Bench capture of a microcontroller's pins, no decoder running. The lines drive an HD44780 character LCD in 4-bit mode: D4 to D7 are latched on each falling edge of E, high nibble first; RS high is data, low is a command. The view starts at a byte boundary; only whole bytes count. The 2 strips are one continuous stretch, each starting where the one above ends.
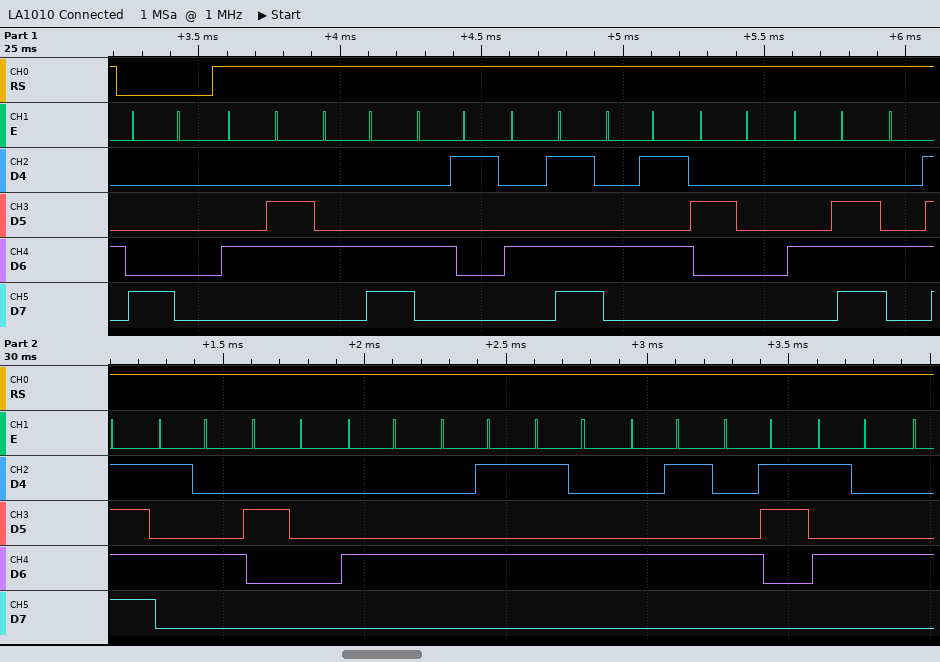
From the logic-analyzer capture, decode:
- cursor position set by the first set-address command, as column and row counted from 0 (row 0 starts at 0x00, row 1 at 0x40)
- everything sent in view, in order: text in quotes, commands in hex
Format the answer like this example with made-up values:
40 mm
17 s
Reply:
column 0, row 0
0x80 "FLAME NOT DETECT"
